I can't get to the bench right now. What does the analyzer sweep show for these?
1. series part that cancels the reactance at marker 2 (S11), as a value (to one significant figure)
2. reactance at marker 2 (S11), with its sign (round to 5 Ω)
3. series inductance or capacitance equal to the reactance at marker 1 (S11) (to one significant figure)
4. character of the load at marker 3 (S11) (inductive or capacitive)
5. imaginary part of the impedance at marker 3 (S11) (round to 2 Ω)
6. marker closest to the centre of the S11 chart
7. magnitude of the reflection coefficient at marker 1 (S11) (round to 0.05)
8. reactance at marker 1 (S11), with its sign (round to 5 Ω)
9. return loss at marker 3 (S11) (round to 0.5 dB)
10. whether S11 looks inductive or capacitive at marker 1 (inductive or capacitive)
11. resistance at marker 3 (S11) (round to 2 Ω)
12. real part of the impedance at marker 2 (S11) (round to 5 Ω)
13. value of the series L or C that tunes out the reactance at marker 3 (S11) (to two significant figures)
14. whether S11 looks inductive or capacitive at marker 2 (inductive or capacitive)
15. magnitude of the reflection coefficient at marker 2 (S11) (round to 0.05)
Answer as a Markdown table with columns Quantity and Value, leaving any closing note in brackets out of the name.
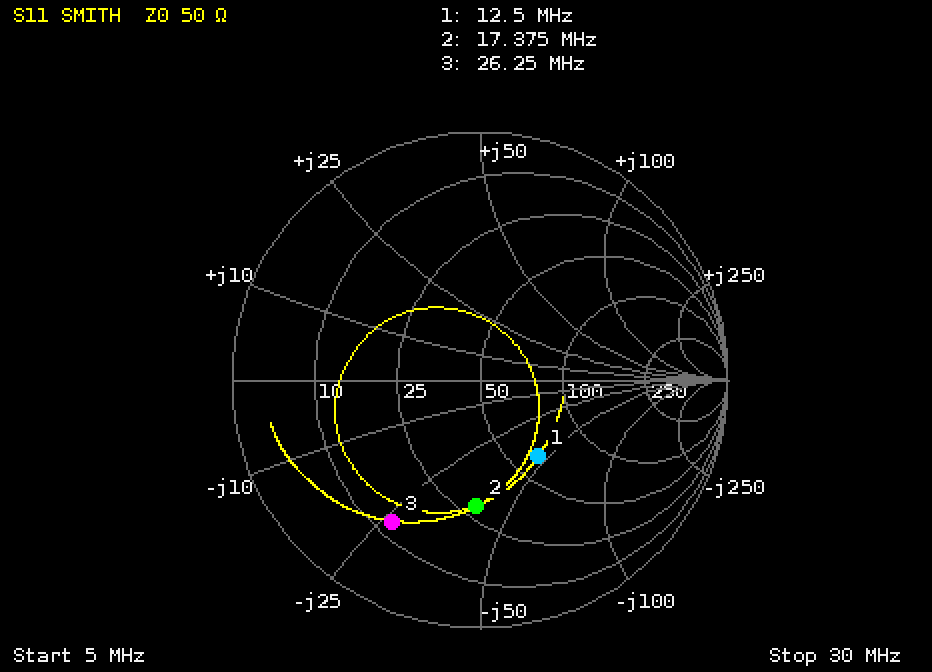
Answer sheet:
| Quantity | Value |
|---|---|
| series part that cancels the reactance at marker 2 (S11), as a value | 400 nH |
| reactance at marker 2 (S11), with its sign | -40 Ω |
| series inductance or capacitance equal to the reactance at marker 1 (S11) | 300 pF |
| character of the load at marker 3 (S11) | capacitive |
| imaginary part of the impedance at marker 3 (S11) | -26 Ω |
| marker closest to the centre of the S11 chart | marker 1 |
| magnitude of the reflection coefficient at marker 1 (S11) | 0.40 |
| reactance at marker 1 (S11), with its sign | -45 Ω |
| return loss at marker 3 (S11) | 3.5 dB |
| whether S11 looks inductive or capacitive at marker 1 | capacitive |
| resistance at marker 3 (S11) | 12 Ω |
| real part of the impedance at marker 2 (S11) | 30 Ω |
| value of the series L or C that tunes out the reactance at marker 3 (S11) | 160 nH |
| whether S11 looks inductive or capacitive at marker 2 | capacitive |
| magnitude of the reflection coefficient at marker 2 (S11) | 0.50 |
